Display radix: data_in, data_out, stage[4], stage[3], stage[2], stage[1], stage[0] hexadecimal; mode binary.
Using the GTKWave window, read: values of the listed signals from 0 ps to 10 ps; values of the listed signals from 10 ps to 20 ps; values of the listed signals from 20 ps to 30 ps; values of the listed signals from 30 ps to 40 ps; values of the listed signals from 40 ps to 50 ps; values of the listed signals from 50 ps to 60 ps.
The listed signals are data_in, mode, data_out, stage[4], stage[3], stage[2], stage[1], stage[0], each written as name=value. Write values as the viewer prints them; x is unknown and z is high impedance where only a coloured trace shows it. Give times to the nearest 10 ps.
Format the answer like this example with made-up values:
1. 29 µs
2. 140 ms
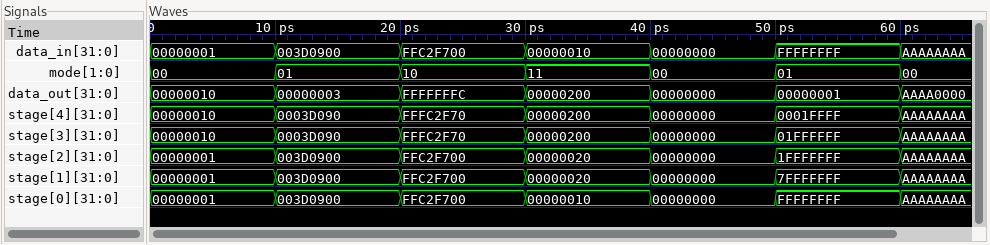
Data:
1. data_in=00000001, mode=00, data_out=00000010, stage[4]=00000010, stage[3]=00000010, stage[2]=00000001, stage[1]=00000001, stage[0]=00000001
2. data_in=003D0900, mode=01, data_out=00000003, stage[4]=0003D090, stage[3]=0003D090, stage[2]=003D0900, stage[1]=003D0900, stage[0]=003D0900
3. data_in=FFC2F700, mode=10, data_out=FFFFFFFC, stage[4]=FFFC2F70, stage[3]=FFFC2F70, stage[2]=FFC2F700, stage[1]=FFC2F700, stage[0]=FFC2F700
4. data_in=00000010, mode=11, data_out=00000200, stage[4]=00000200, stage[3]=00000200, stage[2]=00000020, stage[1]=00000020, stage[0]=00000010
5. data_in=00000000, mode=00, data_out=00000000, stage[4]=00000000, stage[3]=00000000, stage[2]=00000000, stage[1]=00000000, stage[0]=00000000
6. data_in=FFFFFFFF, mode=01, data_out=00000001, stage[4]=0001FFFF, stage[3]=01FFFFFF, stage[2]=1FFFFFFF, stage[1]=7FFFFFFF, stage[0]=FFFFFFFF
